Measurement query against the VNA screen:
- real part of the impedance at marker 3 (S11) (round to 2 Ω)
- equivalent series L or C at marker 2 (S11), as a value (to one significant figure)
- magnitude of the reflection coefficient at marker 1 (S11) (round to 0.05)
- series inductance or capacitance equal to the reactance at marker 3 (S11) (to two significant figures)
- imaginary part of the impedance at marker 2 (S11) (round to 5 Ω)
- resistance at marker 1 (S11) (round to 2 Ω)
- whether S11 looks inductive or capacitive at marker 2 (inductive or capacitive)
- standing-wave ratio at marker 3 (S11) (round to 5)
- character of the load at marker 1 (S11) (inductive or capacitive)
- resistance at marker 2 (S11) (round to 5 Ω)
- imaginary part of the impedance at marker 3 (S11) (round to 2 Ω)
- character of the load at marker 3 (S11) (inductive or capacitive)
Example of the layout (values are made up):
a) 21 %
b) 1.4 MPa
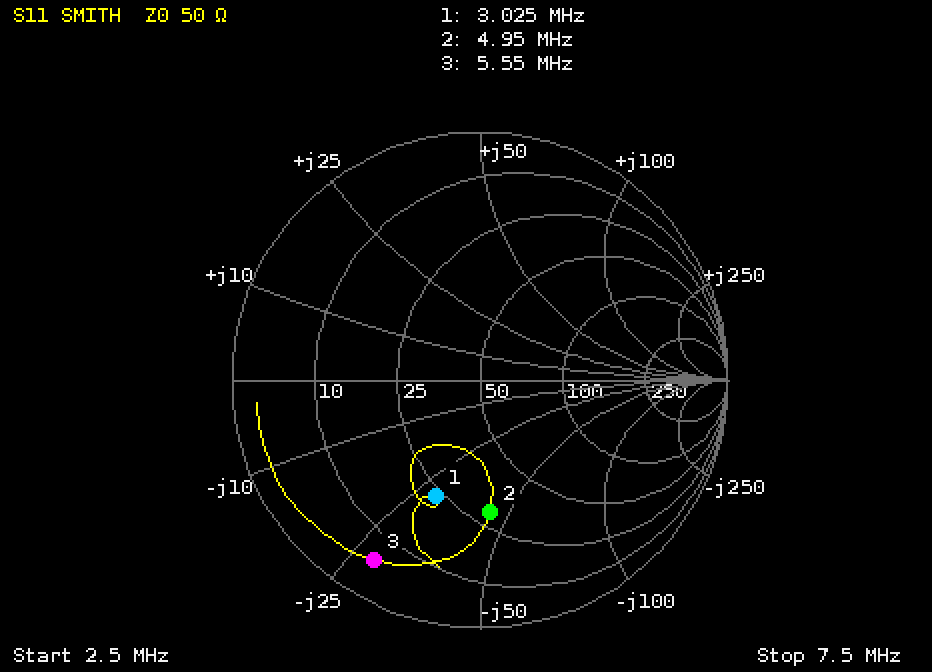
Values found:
a) 6 Ω
b) 700 pF
c) 0.50
d) 1.0 nF
e) -45 Ω
f) 24 Ω
g) capacitive
h) 10
i) capacitive
j) 30 Ω
k) -28 Ω
l) capacitive
